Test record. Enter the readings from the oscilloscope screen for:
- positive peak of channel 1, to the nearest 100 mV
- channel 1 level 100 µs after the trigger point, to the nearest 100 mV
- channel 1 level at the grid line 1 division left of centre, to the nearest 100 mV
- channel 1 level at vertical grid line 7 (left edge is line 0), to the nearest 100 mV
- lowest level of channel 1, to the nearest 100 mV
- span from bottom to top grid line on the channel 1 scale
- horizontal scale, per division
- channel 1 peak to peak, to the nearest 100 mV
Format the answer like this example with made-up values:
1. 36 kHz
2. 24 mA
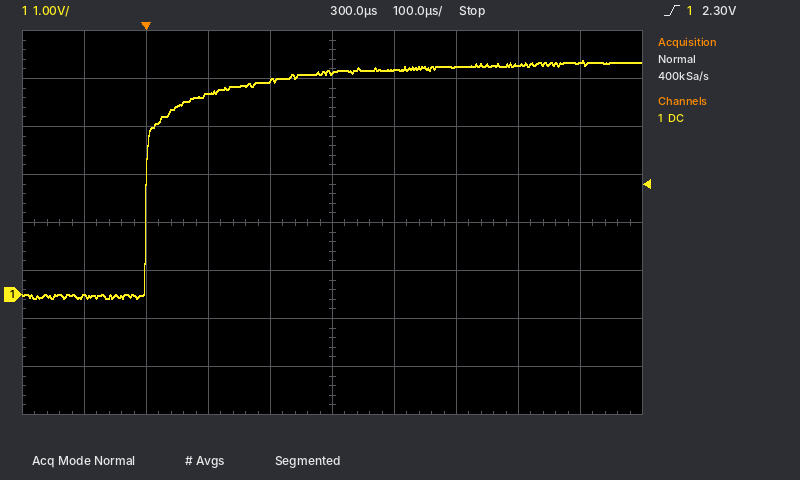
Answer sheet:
1. 4.9 V
2. 4.2 V
3. 4.5 V
4. 4.7 V
5. -100 mV
6. 8 V
7. 100 µs
8. 5.0 V
